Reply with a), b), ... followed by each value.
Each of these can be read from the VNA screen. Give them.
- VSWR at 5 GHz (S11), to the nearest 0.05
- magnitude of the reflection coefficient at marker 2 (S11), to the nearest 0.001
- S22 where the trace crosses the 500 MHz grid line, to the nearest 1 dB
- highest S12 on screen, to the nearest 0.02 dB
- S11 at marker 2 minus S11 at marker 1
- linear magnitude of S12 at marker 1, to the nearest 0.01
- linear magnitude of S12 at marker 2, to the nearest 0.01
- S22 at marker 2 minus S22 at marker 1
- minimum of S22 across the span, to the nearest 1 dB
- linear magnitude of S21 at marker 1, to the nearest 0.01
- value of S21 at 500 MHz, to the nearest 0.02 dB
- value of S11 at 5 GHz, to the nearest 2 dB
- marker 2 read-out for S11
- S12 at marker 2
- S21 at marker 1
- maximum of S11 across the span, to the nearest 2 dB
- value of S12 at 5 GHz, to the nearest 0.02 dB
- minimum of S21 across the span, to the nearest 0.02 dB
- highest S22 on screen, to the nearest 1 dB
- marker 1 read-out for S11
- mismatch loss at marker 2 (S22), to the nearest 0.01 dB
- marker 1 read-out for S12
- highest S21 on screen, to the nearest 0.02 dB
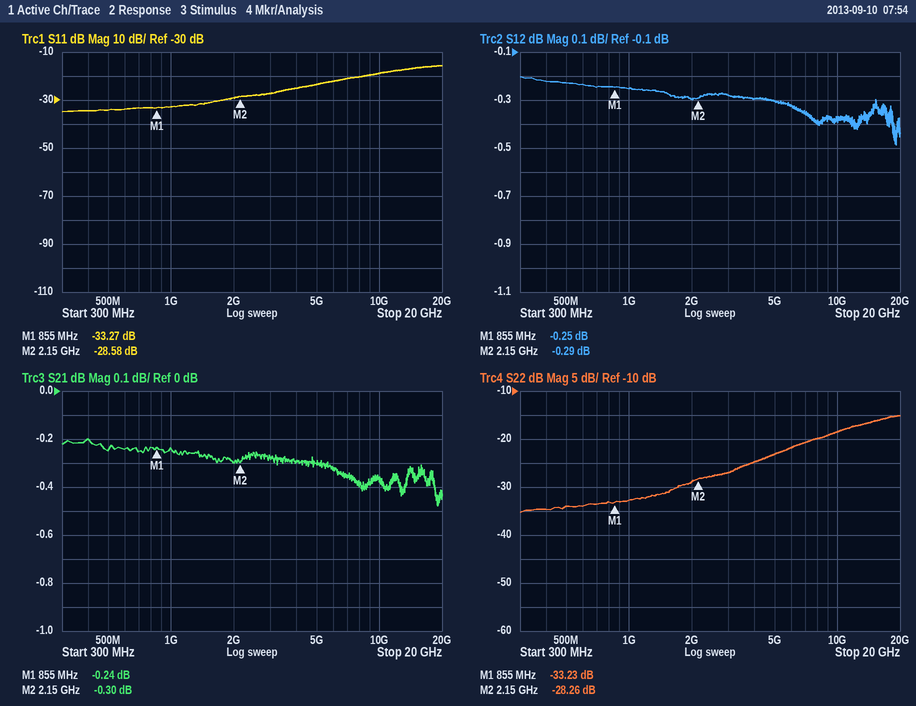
a) 1.15
b) 0.037
c) -34 dB
d) -0.20 dB
e) 4.69 dB
f) 0.97
g) 0.97
h) 4.97 dB
i) -35 dB
j) 0.97
k) -0.24 dB
l) -24 dB
m) -28.58 dB
n) -0.29 dB
o) -0.24 dB
p) -16 dB
q) -0.30 dB
r) -0.48 dB
s) -15 dB
t) -33.27 dB
u) 0.01 dB
v) -0.25 dB
w) -0.20 dB
